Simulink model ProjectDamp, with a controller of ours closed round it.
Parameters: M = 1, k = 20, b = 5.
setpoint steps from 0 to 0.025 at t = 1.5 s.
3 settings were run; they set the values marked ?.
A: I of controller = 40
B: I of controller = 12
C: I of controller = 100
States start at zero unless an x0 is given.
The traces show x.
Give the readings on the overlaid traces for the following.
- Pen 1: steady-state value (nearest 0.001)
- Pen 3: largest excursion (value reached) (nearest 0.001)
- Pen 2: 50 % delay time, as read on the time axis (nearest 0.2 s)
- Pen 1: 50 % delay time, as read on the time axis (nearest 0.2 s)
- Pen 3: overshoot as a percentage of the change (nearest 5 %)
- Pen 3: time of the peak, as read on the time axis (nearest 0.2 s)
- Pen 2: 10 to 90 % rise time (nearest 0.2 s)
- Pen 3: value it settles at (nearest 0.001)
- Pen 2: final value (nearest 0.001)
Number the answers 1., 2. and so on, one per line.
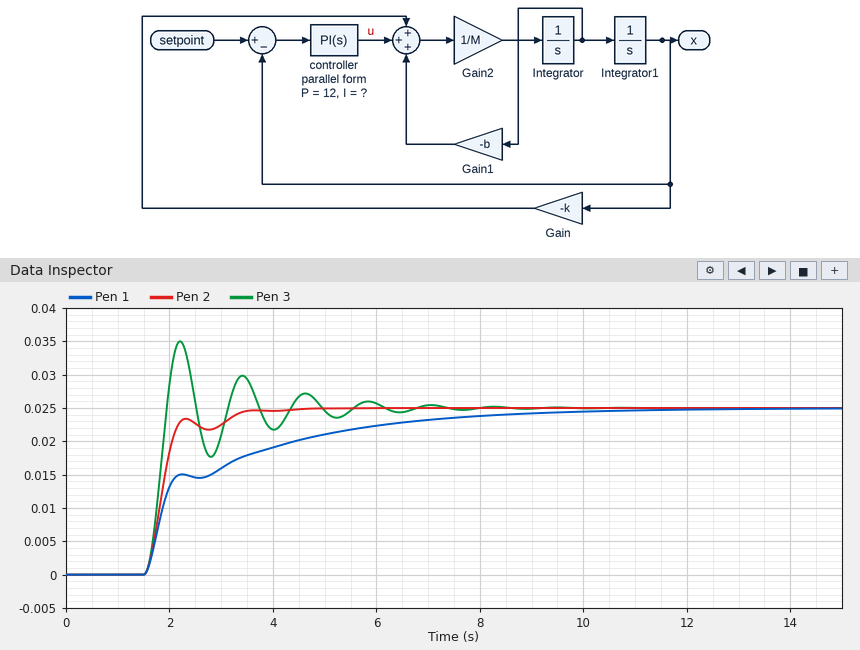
1. 0.025
2. 0.035
3. 1.8 s
4. 2.0 s
5. 40 %
6. 2.2 s
7. 0.6 s
8. 0.025
9. 0.025
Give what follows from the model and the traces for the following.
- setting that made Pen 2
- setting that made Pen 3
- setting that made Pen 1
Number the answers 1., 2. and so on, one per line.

1. A
2. C
3. B
